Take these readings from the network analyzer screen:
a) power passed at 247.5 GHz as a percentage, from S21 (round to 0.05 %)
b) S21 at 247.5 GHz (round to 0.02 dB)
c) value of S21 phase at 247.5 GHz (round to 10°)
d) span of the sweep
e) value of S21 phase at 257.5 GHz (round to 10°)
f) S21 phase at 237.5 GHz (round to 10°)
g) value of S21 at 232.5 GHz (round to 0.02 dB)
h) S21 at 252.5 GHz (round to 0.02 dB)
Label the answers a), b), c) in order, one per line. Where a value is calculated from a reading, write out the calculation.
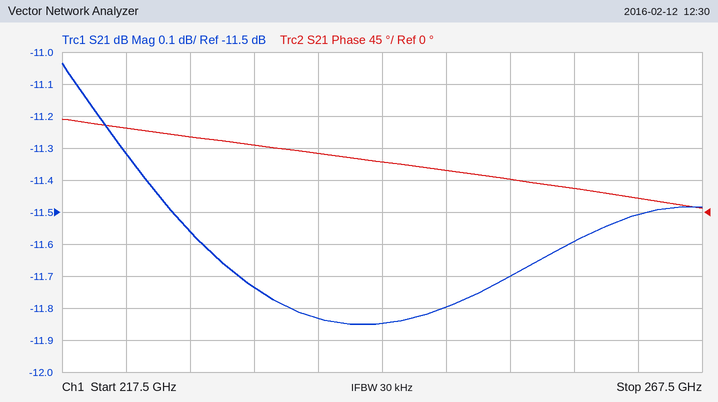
a) 10^(-11.8/10) ≈ 6.61 %, so 6.60 % to the nearest 0.05 %
b) -11.80 dB
c) 60°
d) 50 GHz
e) 30°
f) 80°
g) -11.74 dB
h) -11.70 dB
